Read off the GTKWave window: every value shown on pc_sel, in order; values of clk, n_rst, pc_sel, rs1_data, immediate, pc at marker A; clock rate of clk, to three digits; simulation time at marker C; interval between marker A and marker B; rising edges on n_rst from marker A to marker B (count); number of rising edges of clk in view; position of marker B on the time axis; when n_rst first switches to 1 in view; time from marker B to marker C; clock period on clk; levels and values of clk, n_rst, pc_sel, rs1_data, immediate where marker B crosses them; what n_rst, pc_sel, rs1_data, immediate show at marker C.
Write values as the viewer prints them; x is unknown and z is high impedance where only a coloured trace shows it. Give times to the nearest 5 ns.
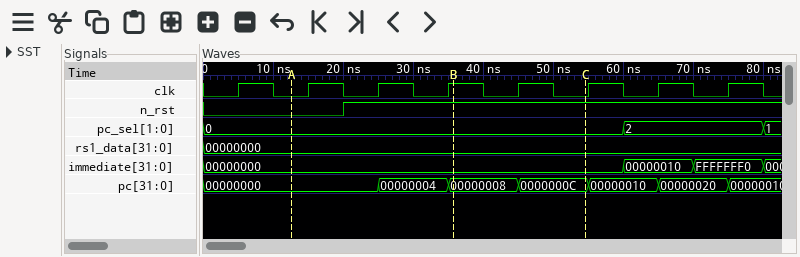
0, 2, 1
clk=0, n_rst=0, pc_sel=0, rs1_data=00000000, immediate=00000000, pc=00000000
100 MHz
55 ns
25 ns
1
8
35 ns
20 ns
20 ns
10 ns
clk=1, n_rst=1, pc_sel=0, rs1_data=00000000, immediate=00000000
n_rst=1, pc_sel=0, rs1_data=00000000, immediate=00000000
